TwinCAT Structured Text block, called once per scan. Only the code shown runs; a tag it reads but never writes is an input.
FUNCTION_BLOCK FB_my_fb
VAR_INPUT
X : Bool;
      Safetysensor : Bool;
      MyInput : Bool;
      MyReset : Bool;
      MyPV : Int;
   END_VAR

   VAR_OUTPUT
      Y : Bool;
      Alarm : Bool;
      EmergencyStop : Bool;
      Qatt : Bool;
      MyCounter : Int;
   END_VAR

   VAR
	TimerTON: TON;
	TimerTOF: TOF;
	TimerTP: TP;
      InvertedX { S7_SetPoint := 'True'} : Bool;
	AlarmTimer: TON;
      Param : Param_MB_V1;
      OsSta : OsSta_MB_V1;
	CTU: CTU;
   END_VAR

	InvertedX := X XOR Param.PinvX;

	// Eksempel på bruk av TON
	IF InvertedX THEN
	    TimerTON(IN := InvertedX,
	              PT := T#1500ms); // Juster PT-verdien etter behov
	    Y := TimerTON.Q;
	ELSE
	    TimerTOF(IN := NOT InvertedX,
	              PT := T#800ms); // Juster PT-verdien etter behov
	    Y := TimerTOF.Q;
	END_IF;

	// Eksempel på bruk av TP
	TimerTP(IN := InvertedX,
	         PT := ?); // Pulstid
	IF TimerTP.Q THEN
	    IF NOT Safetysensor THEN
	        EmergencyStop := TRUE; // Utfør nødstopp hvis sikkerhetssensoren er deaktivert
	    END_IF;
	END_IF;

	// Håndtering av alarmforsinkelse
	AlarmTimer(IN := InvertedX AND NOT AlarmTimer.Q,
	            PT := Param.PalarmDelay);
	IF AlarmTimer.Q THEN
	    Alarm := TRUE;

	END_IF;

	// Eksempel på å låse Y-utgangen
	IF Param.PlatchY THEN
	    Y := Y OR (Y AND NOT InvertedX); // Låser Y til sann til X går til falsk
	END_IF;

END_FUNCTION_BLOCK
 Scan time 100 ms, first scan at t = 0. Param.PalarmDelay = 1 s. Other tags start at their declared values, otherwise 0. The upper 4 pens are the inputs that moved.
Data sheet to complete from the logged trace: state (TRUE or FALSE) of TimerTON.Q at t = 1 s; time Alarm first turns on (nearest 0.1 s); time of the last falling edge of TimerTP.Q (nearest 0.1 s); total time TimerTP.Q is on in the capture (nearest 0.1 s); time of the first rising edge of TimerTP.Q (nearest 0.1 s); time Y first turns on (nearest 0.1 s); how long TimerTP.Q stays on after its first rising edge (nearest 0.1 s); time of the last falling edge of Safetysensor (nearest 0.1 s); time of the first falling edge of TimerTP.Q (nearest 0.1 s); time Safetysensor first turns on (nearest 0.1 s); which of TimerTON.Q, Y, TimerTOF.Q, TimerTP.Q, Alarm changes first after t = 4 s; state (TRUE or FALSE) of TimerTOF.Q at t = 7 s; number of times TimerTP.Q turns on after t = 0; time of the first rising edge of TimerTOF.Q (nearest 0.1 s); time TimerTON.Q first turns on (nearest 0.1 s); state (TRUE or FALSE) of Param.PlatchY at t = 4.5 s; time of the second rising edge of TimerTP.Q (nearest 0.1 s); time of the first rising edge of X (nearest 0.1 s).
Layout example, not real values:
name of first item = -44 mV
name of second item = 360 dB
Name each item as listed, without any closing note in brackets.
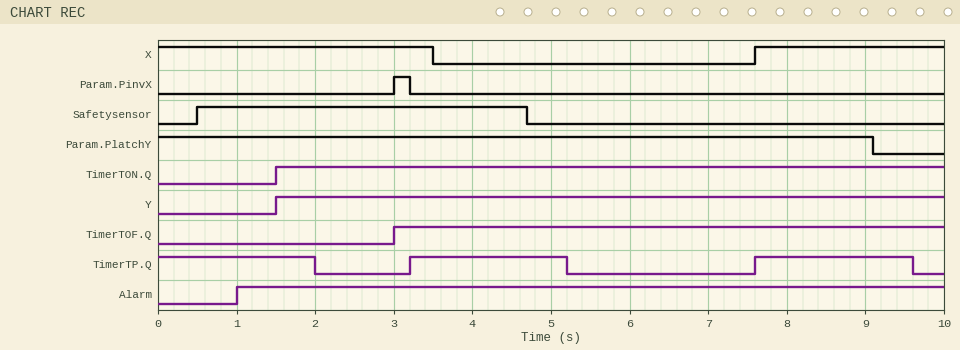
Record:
state (TRUE or FALSE) of TimerTON.Q at t = 1 s = FALSE
time Alarm first turns on = 1.0 s
time of the last falling edge of TimerTP.Q = 9.6 s
total time TimerTP.Q is on in the capture = 6.0 s
time of the first rising edge of TimerTP.Q = 3.2 s
time Y first turns on = 1.5 s
how long TimerTP.Q stays on after its first rising edge = 2.0 s
time of the last falling edge of Safetysensor = 4.7 s
time of the first falling edge of TimerTP.Q = 2.0 s
time Safetysensor first turns on = 0.5 s
which of TimerTON.Q, Y, TimerTOF.Q, TimerTP.Q, Alarm changes first after t = 4 s = TimerTP.Q
state (TRUE or FALSE) of TimerTOF.Q at t = 7 s = TRUE
number of times TimerTP.Q turns on after t = 0 = 2
time of the first rising edge of TimerTOF.Q = 3.0 s
time TimerTON.Q first turns on = 1.5 s
state (TRUE or FALSE) of Param.PlatchY at t = 4.5 s = TRUE
time of the second rising edge of TimerTP.Q = 7.6 s
time of the first rising edge of X = 7.6 s
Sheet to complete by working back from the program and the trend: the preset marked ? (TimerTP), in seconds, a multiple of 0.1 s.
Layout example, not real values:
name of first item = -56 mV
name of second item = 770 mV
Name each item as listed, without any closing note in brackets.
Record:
the preset marked ? (TimerTP), in seconds, a multiple of 0.1 s = 2.0 s
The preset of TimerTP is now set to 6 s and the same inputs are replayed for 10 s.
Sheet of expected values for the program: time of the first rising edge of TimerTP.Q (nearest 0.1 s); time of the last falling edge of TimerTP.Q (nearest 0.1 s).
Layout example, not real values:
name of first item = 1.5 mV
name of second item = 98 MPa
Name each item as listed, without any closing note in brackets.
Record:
time of the first rising edge of TimerTP.Q = 7.6 s
time of the last falling edge of TimerTP.Q = 6.0 s
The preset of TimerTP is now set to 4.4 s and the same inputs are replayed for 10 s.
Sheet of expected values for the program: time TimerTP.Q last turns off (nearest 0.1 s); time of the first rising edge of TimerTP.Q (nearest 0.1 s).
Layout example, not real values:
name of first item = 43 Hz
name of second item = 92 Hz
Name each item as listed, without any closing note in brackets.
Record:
time TimerTP.Q last turns off = 4.4 s
time of the first rising edge of TimerTP.Q = 7.6 s
